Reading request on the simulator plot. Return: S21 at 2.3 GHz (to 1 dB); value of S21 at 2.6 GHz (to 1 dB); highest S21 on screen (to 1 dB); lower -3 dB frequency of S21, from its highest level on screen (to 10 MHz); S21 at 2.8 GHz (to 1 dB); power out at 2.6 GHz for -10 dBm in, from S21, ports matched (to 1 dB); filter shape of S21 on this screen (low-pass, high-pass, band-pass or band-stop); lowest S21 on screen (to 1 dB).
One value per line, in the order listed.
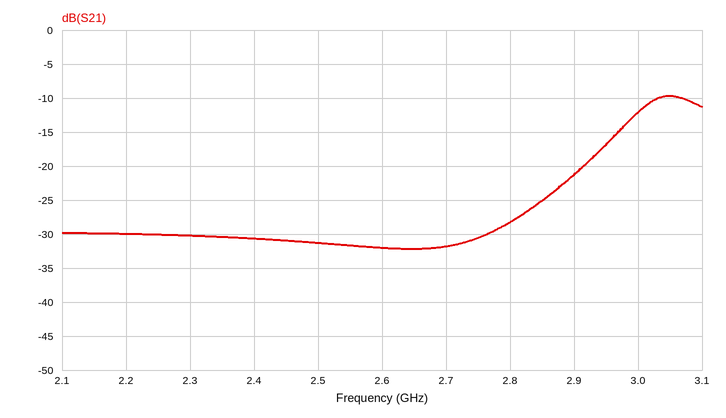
-30 dB
-32 dB
-10 dB
2.99 GHz
-28 dB
-42 dBm
high-pass
-32 dB
